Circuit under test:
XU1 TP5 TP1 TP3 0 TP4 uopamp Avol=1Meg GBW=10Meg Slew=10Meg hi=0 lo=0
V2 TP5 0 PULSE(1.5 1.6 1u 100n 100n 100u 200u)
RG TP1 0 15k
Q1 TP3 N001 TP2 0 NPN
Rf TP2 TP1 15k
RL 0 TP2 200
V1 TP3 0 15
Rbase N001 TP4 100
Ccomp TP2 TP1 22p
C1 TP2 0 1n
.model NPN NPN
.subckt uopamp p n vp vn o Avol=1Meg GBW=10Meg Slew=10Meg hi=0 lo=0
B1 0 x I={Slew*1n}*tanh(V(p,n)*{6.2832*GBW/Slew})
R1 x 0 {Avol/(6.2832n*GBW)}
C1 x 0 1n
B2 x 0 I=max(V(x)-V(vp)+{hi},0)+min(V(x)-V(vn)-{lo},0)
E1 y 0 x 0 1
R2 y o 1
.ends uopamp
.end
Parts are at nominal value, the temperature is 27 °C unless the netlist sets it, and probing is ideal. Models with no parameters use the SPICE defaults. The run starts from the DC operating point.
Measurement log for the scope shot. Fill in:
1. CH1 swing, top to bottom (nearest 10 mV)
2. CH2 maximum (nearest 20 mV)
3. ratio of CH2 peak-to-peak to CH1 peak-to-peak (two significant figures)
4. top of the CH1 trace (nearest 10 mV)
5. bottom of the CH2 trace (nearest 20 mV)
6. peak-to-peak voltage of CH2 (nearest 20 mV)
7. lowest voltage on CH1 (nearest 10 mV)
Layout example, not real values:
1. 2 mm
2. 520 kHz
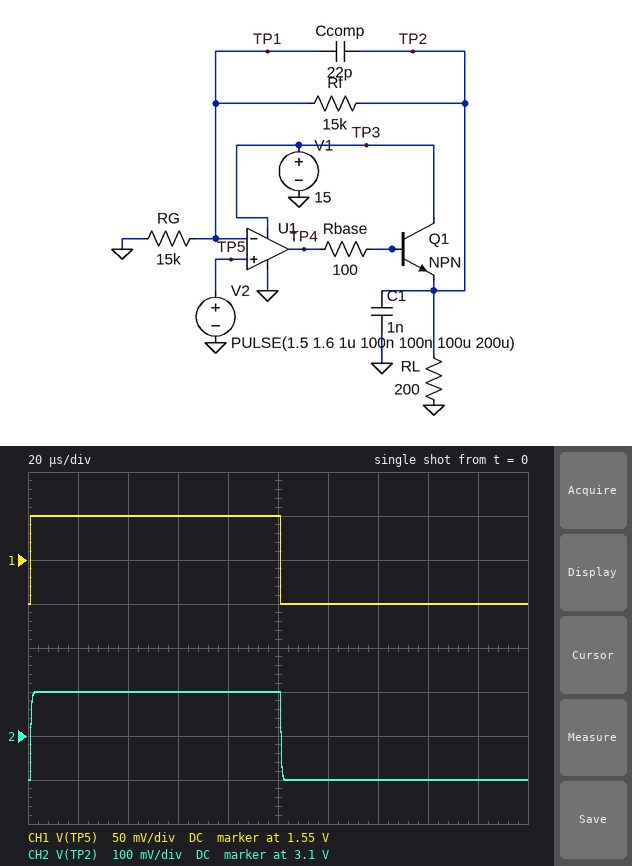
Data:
1. 100 mV
2. 3.20 V
3. 2.0
4. 1.60 V
5. 3.00 V
6. 200 mV
7. 1.50 V
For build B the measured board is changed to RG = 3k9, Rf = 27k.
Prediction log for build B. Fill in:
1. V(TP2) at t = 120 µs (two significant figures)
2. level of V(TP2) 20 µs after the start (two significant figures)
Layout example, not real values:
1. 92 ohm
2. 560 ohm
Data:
1. 12 V
2. 13 V
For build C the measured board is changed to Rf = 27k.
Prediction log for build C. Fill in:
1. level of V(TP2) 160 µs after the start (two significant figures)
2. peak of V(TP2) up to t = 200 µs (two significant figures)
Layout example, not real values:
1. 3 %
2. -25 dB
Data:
1. 4.2 V
2. 4.5 V
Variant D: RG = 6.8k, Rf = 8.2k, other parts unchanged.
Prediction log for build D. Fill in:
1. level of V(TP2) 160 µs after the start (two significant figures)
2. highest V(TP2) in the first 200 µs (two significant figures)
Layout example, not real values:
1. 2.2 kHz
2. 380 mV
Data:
1. 3.3 V
2. 3.5 V
